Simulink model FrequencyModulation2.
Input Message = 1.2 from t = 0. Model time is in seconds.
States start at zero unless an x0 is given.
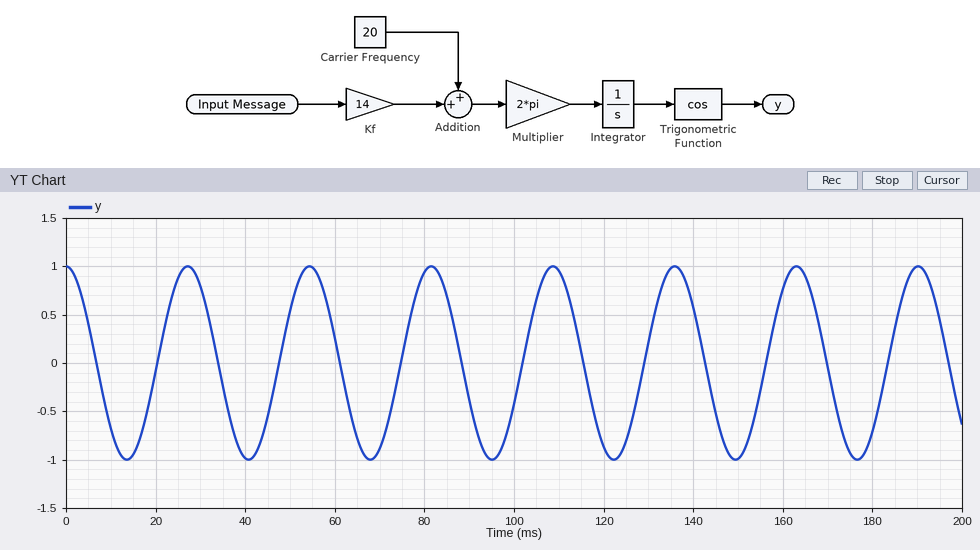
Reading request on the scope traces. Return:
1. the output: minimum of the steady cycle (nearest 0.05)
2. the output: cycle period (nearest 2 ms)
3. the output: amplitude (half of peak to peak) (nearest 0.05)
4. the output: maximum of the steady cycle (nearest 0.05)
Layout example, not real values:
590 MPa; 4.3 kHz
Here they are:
-1.00; 28 ms; 1.00; 1.00
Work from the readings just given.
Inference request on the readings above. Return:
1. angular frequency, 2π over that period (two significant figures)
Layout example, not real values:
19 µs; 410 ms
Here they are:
0.22 rad/ms
